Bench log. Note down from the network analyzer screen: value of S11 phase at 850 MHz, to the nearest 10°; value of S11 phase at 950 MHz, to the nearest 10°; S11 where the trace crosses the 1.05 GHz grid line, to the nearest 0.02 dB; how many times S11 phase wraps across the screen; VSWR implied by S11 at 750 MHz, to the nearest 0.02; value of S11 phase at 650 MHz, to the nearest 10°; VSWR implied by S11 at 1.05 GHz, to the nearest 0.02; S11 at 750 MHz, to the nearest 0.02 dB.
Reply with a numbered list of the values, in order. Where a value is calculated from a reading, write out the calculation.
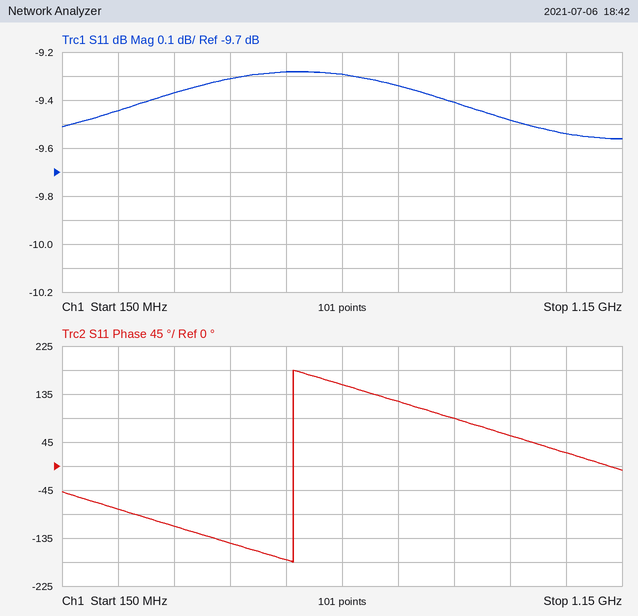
1. 90°
2. 60°
3. -9.54 dB
4. 1
5. |Γ| = 10^(-9.34/20) = 0.3412; VSWR = (1 + 0.3412)/(1 − 0.3412) ≈ 2.04
6. 150°
7. |Γ| = 10^(-9.54/20) = 0.3334; VSWR = (1 + 0.3334)/(1 − 0.3334) ≈ 2.00
8. -9.34 dB
